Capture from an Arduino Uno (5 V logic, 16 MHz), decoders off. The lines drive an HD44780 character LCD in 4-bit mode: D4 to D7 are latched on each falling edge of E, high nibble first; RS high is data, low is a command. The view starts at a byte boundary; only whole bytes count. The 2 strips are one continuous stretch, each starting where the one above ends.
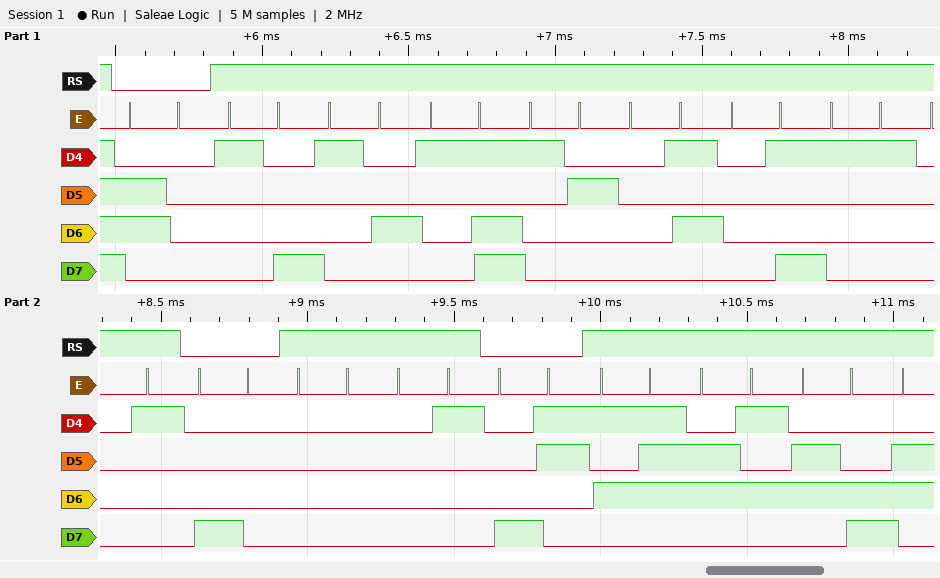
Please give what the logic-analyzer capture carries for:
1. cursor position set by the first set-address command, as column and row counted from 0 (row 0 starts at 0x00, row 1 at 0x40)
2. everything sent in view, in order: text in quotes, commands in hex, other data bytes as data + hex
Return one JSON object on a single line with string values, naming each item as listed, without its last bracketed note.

{"cursor position set by the first set-address command, as column and row counted from 0": "column 0, row 0", "everything sent in view, in order: text in quotes, commands in hex, other data bytes as data + hex": "0x60 data 18 14 1D 12 05 09 11 01 0x80 data 00 01 0x83 \"Wel\""}
